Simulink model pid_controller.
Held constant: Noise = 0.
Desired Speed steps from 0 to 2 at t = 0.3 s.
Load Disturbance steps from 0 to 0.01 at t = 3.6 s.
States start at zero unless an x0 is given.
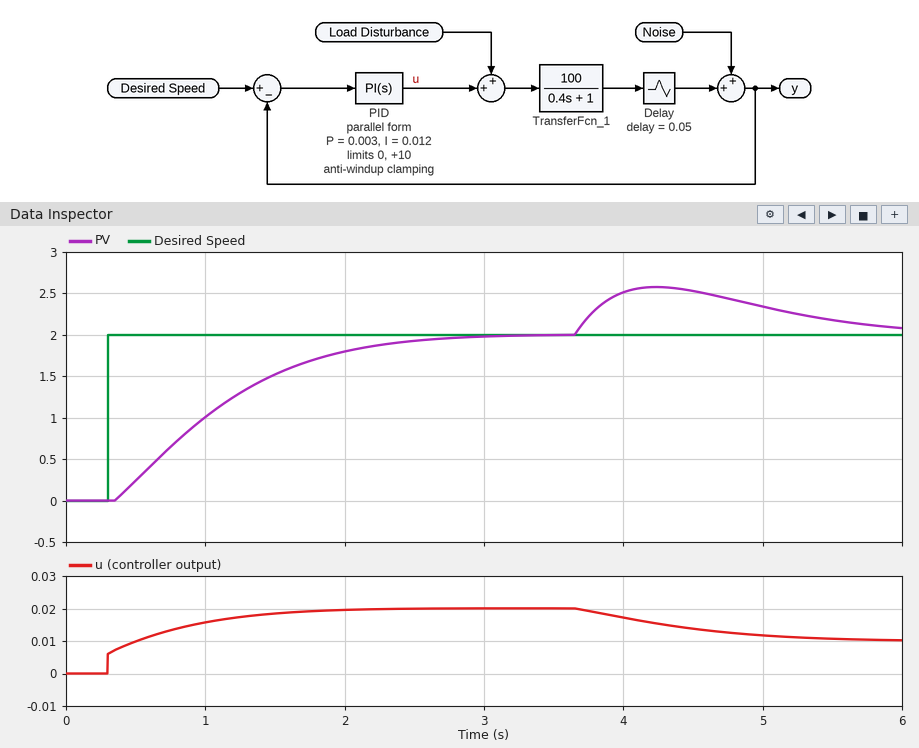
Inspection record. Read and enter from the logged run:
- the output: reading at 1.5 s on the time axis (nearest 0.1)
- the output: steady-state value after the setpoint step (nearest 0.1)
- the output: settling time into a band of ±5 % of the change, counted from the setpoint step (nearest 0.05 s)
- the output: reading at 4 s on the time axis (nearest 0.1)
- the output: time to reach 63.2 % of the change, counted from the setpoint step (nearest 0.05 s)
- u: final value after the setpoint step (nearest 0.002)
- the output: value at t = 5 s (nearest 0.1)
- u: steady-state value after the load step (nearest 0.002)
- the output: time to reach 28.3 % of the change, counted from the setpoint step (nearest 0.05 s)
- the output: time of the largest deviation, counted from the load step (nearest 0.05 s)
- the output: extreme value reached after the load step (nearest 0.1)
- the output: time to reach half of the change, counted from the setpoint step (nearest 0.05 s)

1.5
2.0
2.05 s
2.5
0.90 s
0.020
2.3
0.010
0.40 s
0.65 s
2.6
0.70 s
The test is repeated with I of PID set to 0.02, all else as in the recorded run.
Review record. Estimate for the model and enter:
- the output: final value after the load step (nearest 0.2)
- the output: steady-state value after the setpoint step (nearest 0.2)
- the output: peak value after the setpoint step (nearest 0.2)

2.0
2.0
2.2
